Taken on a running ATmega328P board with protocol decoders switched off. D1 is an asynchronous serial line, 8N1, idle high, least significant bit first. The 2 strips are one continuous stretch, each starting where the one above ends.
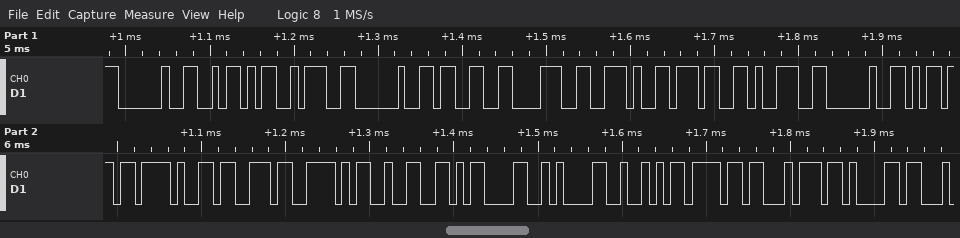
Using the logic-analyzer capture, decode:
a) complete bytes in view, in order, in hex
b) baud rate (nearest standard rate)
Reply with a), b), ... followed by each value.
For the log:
a) 0x20 0x5A 0x3A 0x20 0x33 0x38 0x2E 0x37 0x39 0x20 0x6D 0x2F 0x73 0x5E 0x32 0x0D 0x0A 0x52 0x6F 0x74 0x61
b) 115200 baud
